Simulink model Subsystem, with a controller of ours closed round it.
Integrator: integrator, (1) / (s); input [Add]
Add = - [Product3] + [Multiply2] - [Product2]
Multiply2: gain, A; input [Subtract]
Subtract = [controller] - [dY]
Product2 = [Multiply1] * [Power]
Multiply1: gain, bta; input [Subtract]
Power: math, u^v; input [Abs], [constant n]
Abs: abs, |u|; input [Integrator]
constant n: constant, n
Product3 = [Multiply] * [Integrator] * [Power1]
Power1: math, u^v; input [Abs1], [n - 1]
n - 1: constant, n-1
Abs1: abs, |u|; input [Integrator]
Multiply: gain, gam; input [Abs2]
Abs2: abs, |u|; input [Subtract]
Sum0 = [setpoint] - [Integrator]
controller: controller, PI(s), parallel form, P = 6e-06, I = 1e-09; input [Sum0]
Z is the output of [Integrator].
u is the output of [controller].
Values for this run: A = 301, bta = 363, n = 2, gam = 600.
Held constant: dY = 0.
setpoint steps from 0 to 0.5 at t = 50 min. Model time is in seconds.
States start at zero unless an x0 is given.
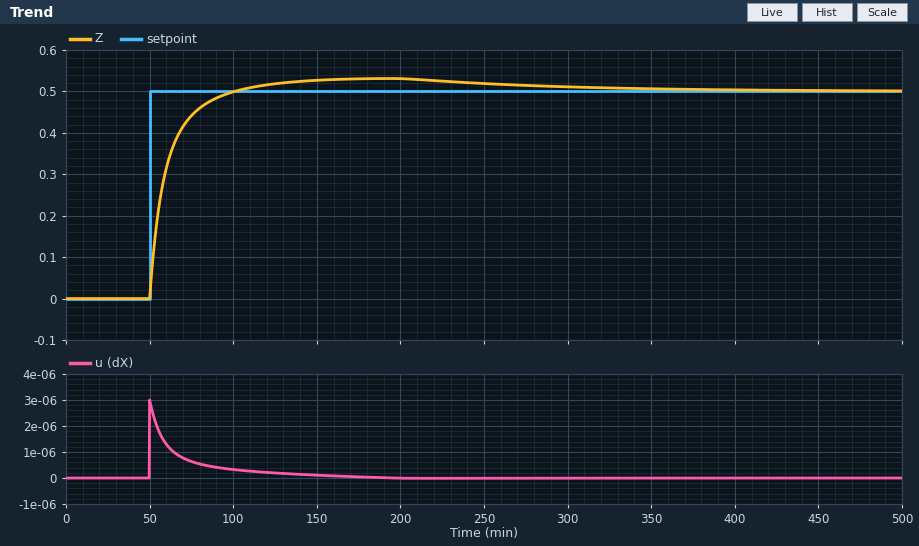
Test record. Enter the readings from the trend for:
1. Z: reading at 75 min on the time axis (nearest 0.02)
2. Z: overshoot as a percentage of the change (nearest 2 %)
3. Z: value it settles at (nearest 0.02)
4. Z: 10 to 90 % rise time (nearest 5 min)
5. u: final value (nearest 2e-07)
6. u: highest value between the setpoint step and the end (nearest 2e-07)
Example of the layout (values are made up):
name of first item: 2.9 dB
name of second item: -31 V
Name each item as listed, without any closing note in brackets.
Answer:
Z: reading at 75 min on the time axis: 0.44
Z: overshoot as a percentage of the change: 6 %
Z: value it settles at: 0.50
Z: 10 to 90 % rise time: 25 min
u: final value: 0.0000000
u: highest value between the setpoint step and the end: 0.0000030
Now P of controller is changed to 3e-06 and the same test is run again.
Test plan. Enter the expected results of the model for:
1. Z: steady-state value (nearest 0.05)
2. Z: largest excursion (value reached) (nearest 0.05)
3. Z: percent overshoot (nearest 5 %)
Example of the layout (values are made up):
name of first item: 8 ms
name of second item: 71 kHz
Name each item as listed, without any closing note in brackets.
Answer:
Z: steady-state value: 0.50
Z: largest excursion (value reached): 0.55
Z: percent overshoot: 10 %
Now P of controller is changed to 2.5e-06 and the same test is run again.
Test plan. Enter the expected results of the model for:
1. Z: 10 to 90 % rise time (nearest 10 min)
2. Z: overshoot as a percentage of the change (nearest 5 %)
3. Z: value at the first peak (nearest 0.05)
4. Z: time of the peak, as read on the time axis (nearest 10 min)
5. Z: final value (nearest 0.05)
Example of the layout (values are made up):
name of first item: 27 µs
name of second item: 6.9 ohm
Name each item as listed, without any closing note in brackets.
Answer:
Z: 10 to 90 % rise time: 40 min
Z: overshoot as a percentage of the change: 10 %
Z: value at the first peak: 0.55
Z: time of the peak, as read on the time axis: 260 min
Z: final value: 0.50
